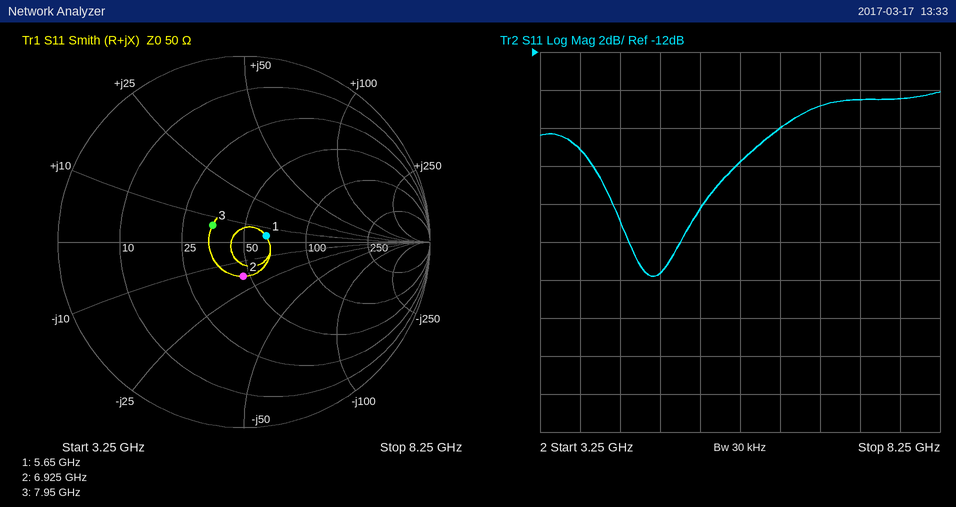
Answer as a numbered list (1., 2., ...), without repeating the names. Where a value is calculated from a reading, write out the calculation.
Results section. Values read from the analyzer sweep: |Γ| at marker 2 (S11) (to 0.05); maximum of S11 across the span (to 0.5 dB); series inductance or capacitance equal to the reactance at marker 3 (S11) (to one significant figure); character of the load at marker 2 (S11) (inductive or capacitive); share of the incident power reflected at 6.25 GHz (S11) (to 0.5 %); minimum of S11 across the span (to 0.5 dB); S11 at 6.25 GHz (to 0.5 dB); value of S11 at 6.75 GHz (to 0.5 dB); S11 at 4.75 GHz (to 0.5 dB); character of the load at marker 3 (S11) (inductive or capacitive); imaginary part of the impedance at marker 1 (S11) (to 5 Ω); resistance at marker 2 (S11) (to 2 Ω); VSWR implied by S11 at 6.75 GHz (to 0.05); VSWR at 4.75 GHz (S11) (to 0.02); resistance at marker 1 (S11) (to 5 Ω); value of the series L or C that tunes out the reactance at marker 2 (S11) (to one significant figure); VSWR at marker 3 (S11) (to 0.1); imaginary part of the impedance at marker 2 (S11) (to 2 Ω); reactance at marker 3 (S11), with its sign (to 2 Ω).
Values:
1. 0.20
2. -14.0 dB
3. L = 6 Ω/(2π × 7.95 GHz) ≈ 120 pH, so 100 pH to one significant figure
4. capacitive
5. 10^(-16/10) ≈ 2.5 %
6. -24.0 dB
7. -16.0 dB
8. -15.0 dB
9. -23.5 dB
10. inductive
11. +5 Ω
12. 46 Ω
13. |Γ| = 10^(-15/20) = 0.1778; VSWR = (1 + 0.1778)/(1 − 0.1778) ≈ 1.43, so 1.45 to the nearest 0.05
14. |Γ| = 10^(-23.5/20) = 0.0668; VSWR = (1 + 0.0668)/(1 − 0.0668) ≈ 1.14
15. 65 Ω
16. L = 18 Ω/(2π × 6.925 GHz) ≈ 414 pH, so 400 pH to one significant figure
17. 1.5
18. -18 Ω
19. +6 Ω
